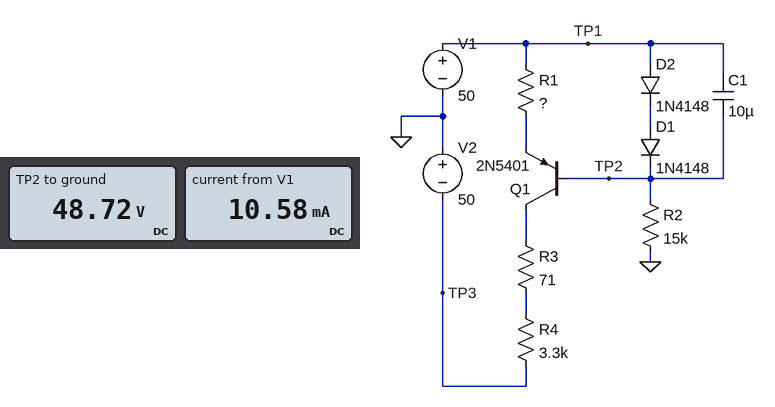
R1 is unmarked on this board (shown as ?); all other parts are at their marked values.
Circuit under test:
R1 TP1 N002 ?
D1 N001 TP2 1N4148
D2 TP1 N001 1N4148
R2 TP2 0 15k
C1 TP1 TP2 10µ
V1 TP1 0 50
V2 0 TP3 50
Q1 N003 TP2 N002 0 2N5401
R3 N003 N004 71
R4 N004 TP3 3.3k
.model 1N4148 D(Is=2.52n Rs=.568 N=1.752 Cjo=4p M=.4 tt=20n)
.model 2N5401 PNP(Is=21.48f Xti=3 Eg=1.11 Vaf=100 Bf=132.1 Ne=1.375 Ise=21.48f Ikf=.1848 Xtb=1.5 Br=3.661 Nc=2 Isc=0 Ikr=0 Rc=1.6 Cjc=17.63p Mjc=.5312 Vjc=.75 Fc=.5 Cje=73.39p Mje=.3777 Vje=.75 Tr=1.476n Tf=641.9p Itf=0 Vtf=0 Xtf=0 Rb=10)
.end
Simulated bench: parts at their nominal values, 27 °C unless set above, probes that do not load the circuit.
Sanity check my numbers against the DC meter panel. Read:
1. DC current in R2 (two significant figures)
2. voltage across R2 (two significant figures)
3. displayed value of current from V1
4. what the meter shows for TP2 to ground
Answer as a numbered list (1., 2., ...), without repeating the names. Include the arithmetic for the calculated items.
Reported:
1. (48.72 V) / 15 kΩ = 3.2 mA
2. 48.72 V = 49 V
3. 10.58 mA
4. 48.72 V
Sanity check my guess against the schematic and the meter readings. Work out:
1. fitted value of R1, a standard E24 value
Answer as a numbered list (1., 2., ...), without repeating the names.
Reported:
1. 82 Ω
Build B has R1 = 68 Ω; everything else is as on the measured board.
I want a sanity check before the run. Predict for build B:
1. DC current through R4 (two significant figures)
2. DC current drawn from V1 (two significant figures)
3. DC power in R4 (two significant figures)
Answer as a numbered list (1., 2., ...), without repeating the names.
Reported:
1. 8.8 mA
2. 12 mA
3. 250 mW
